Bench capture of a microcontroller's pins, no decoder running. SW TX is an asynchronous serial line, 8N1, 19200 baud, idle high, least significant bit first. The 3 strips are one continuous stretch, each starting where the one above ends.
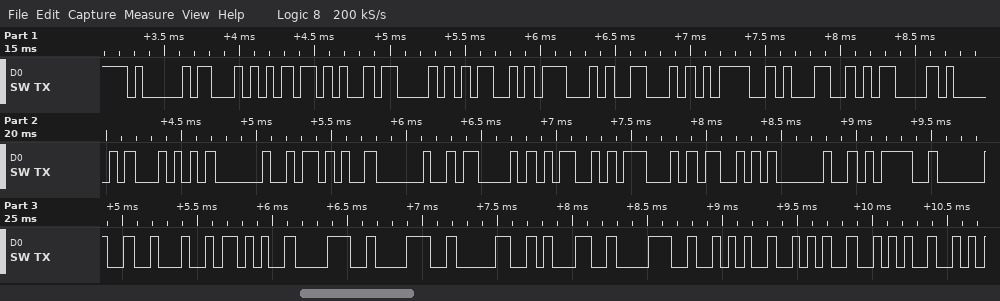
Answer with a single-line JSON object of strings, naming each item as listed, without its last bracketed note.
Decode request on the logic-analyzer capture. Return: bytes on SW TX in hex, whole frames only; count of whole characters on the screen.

{"bytes on SW TX in hex, whole frames only": "41 54 2B 43 4D 47 46 3D 31 0D 41 54 20 2B 20 43 4D 47 53 20 3D 20 22 2B 38 38 30 31 38 2A 2A 2A", "count of whole characters on the screen": "32"}
